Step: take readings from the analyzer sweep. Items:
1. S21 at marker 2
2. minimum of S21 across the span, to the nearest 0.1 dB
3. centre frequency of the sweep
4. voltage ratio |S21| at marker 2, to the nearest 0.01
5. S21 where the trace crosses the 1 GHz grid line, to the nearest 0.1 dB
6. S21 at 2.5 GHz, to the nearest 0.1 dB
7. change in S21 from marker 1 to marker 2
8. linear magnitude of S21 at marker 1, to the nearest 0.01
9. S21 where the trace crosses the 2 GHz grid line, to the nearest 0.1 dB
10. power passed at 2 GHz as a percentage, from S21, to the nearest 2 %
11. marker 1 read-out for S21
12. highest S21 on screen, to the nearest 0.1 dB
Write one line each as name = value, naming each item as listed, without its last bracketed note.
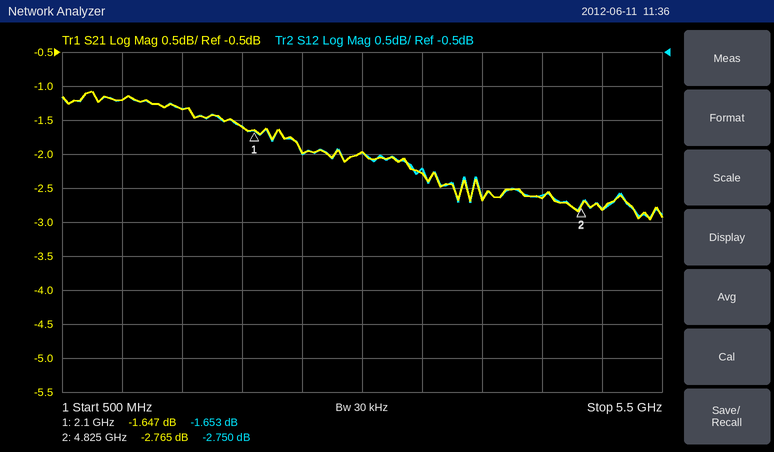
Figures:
S21 at marker 2 = -2.765 dB
minimum of S21 across the span, to the nearest 0.1 dB = -3.0 dB
centre frequency of the sweep = 3 GHz
voltage ratio |S21| at marker 2, to the nearest 0.01 = 0.73
S21 where the trace crosses the 1 GHz grid line, to the nearest 0.1 dB = -1.2 dB
S21 at 2.5 GHz, to the nearest 0.1 dB = -2.0 dB
change in S21 from marker 1 to marker 2 = -1.118 dB
linear magnitude of S21 at marker 1, to the nearest 0.01 = 0.83
S21 where the trace crosses the 2 GHz grid line, to the nearest 0.1 dB = -1.6 dB
power passed at 2 GHz as a percentage, from S21, to the nearest 2 % = 70 %
marker 1 read-out for S21 = -1.647 dB
highest S21 on screen, to the nearest 0.1 dB = -1.1 dB
